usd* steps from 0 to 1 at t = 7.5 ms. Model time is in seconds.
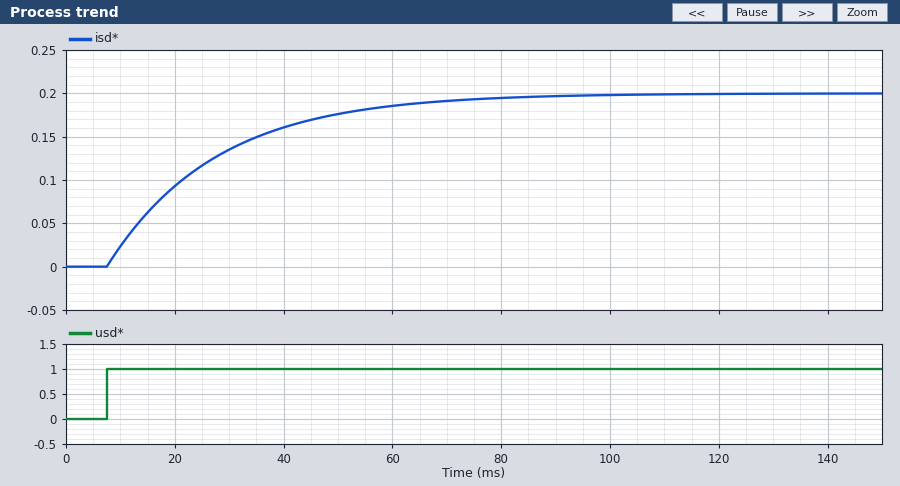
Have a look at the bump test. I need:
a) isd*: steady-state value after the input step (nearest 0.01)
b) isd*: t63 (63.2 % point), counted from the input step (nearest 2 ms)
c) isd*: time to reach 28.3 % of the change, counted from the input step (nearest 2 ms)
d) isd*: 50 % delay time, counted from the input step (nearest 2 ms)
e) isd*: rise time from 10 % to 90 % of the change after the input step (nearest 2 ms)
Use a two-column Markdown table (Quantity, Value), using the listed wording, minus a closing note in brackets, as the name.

| Quantity | Value |
|---|---|
| isd*: steady-state value after the input step | 0.20 |
| isd*: t63 (63.2 % point), counted from the input step | 20 ms |
| isd*: time to reach 28.3 % of the change, counted from the input step | 6 ms |
| isd*: 50 % delay time, counted from the input step | 14 ms |
| isd*: rise time from 10 % to 90 % of the change after the input step | 44 ms |
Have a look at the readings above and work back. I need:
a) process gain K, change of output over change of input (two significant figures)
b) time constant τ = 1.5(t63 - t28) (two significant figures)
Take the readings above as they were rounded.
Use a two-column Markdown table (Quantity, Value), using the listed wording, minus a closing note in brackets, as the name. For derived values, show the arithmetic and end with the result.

| Quantity | Value |
|---|---|
| process gain K, change of output over change of input | (0.2 - 0) / 1 = 0.20 |
| time constant τ = 1.5(t63 - t28) | 1.5 × (20 - 6) = 21 ms |
